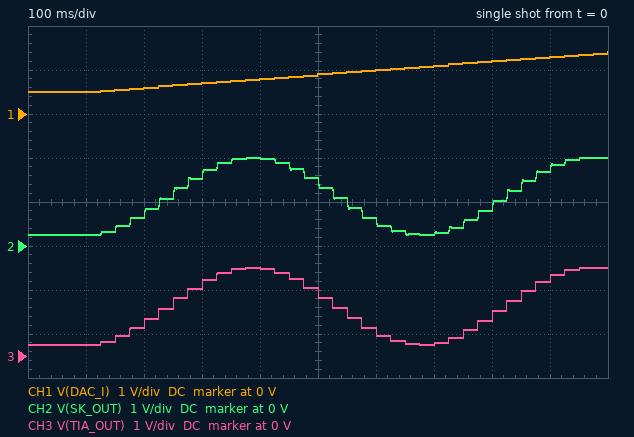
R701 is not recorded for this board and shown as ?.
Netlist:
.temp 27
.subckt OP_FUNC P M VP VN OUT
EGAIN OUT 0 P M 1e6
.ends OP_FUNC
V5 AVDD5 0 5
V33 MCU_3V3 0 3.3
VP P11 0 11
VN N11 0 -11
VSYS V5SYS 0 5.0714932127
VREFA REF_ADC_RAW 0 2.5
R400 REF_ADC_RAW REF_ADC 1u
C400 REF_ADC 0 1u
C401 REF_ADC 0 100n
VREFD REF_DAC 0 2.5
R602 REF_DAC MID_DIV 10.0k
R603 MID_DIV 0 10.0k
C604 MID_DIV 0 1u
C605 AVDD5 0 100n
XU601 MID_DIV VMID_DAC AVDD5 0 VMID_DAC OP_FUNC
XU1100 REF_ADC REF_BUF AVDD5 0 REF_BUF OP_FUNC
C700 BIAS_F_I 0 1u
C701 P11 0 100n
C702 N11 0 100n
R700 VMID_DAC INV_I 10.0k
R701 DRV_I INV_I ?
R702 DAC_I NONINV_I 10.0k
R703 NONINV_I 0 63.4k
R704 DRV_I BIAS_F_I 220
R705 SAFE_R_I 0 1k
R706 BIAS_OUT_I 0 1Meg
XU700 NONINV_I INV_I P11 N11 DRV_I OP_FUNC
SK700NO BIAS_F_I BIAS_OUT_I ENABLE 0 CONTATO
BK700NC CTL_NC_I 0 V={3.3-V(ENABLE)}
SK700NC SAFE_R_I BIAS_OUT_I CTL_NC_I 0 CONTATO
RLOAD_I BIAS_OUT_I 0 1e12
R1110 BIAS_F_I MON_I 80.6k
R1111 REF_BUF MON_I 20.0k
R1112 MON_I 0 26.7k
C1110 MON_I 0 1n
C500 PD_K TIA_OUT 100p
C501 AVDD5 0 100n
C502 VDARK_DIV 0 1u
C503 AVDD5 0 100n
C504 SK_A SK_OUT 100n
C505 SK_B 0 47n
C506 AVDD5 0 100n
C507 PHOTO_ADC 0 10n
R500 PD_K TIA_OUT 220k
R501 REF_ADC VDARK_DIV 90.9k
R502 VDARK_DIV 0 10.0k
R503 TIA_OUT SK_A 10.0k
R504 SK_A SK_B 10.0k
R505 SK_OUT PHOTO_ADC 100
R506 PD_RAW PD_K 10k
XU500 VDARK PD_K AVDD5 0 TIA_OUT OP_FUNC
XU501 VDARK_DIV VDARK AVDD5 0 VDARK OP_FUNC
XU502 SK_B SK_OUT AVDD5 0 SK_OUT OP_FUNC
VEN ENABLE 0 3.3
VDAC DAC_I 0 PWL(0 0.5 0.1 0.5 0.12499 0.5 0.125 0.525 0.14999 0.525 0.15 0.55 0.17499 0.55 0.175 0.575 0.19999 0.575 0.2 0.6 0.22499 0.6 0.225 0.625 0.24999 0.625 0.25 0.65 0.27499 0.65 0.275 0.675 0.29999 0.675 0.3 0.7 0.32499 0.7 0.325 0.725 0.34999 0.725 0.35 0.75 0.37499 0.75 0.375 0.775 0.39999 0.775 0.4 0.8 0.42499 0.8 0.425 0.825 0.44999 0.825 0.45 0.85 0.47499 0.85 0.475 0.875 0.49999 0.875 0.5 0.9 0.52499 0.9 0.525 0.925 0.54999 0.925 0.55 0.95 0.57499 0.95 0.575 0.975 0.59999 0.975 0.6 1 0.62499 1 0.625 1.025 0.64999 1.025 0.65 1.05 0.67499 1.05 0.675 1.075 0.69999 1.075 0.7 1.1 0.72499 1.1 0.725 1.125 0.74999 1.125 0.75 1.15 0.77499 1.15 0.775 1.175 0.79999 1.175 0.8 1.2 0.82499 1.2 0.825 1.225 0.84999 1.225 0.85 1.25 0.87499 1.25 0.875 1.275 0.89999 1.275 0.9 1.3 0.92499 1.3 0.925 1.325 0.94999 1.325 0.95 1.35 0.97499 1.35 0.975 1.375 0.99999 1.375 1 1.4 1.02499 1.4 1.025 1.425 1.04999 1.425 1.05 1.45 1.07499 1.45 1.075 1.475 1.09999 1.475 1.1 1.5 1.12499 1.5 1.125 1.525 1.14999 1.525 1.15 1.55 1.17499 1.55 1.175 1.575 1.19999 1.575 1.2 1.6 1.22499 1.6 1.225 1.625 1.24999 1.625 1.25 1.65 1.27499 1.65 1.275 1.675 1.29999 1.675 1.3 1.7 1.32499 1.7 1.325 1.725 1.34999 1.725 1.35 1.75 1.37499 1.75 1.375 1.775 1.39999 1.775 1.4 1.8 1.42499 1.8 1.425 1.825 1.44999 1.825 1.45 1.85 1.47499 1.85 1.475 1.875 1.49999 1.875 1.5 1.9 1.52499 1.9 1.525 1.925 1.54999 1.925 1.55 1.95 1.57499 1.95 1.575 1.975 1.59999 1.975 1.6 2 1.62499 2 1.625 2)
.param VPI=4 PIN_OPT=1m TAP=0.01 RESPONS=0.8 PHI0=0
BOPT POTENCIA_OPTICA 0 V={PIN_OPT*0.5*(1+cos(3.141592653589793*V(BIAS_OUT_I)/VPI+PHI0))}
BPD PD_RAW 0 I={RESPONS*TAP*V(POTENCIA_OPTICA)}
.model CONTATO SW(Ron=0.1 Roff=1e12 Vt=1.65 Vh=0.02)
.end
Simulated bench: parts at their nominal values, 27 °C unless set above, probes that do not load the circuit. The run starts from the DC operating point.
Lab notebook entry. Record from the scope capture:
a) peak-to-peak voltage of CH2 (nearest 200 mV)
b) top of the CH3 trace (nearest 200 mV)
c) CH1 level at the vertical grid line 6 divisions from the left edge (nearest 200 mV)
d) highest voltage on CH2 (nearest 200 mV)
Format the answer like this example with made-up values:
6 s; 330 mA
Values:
1.8 V; 2.0 V; 1.0 V; 2.0 V
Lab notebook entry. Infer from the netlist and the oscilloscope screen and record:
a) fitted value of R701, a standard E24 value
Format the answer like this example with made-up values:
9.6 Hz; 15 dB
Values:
150 kΩ
